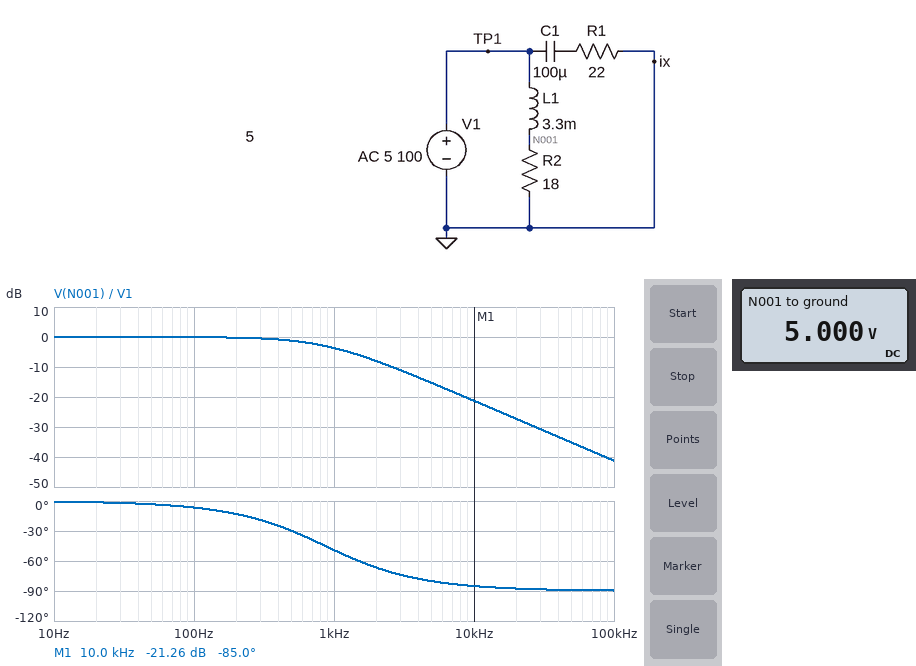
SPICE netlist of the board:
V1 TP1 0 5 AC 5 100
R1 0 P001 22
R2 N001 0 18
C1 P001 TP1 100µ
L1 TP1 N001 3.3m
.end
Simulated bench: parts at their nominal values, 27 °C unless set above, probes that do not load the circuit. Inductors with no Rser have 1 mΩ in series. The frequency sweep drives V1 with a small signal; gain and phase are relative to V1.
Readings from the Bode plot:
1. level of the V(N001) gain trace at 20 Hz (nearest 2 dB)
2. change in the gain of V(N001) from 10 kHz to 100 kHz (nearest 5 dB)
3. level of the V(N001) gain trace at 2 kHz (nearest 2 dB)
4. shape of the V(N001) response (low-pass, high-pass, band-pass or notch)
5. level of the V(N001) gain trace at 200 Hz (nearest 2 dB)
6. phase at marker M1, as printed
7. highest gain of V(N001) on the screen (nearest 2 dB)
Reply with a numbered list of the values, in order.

1. 0 dB
2. -20 dB
3. -8 dB
4. low-pass
5. 0 dB
6. -85.0 deg
7. 0 dB
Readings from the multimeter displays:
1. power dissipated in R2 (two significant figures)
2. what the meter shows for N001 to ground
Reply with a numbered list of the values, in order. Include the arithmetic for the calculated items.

1. (5 V)^2 / 18 Ω = 1.4 W
2. 5.000 V
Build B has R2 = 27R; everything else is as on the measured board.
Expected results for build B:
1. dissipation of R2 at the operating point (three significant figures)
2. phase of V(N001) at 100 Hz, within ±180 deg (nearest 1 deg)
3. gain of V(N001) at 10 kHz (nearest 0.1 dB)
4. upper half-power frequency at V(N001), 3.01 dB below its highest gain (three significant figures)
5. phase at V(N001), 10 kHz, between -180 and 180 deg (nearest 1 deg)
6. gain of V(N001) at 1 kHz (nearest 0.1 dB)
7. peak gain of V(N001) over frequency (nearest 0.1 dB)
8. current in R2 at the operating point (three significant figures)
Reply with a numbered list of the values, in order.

1. 926 mW
2. -4 deg
3. -17.8 dB
4. 1.30 kHz
5. -83 deg
6. -2.0 dB
7. 0 dB
8. 185 mA
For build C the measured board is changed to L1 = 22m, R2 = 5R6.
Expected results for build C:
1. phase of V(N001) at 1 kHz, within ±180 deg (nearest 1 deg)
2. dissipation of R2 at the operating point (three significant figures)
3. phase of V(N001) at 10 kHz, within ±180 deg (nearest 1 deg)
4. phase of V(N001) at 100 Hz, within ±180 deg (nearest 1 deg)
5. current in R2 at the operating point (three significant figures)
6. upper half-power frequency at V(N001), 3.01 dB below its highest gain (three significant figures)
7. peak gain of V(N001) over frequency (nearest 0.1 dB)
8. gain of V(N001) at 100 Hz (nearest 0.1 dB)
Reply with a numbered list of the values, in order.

1. -88 deg
2. 4.46 W
3. -90 deg
4. -68 deg
5. 893 mA
6. 40.5 Hz
7. 0 dB
8. -8.5 dB
